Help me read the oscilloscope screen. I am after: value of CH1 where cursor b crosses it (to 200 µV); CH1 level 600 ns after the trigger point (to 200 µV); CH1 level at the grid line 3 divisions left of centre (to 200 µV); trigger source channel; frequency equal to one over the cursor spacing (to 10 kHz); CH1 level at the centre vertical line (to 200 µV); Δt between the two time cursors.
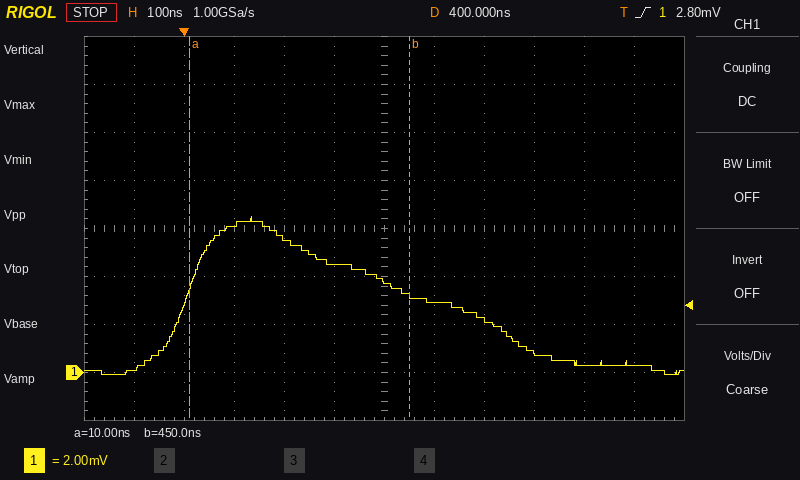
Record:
3.2 mV
2.2 mV
6.2 mV
CH1
2.27 MHz
3.8 mV
440 ns
